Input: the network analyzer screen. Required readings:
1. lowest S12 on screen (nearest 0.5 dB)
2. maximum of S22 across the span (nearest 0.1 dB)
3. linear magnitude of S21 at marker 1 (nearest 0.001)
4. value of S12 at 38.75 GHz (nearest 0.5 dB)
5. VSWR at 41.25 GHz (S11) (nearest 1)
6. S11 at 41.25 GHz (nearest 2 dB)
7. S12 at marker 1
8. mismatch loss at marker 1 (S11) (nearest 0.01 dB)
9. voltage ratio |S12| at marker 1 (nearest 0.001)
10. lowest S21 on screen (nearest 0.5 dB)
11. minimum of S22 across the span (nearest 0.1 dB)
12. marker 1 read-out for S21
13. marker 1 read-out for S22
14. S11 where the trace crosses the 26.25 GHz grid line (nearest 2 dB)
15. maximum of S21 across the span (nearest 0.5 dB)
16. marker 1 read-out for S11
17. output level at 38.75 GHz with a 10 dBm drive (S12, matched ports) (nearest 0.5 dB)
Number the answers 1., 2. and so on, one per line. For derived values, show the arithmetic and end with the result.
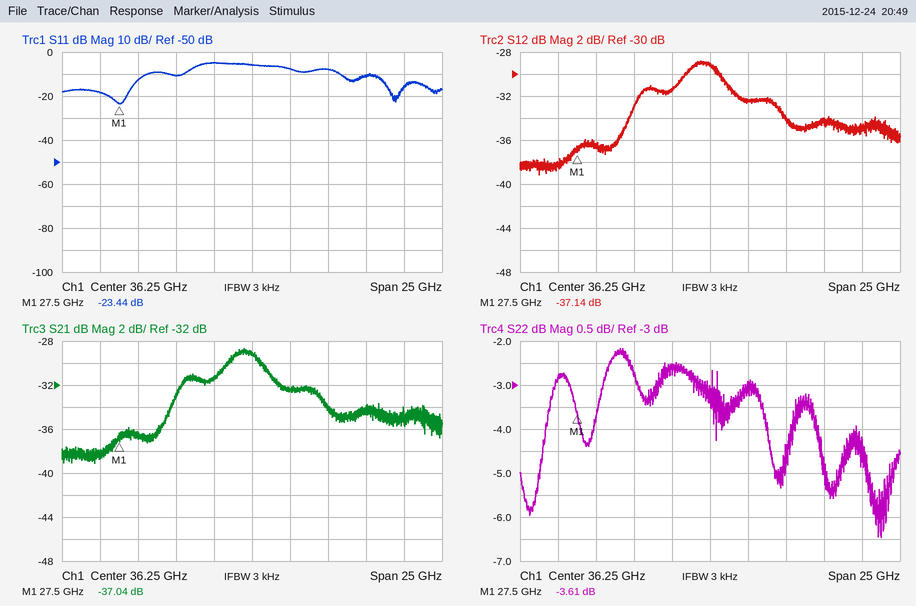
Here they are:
1. -39.0 dB
2. -2.2 dB
3. 10^(-37.04/20) ≈ 0.014
4. -32.5 dB
5. |Γ| = 10^(-8/20) = 0.3981; VSWR = (1 + 0.3981)/(1 − 0.3981) ≈ 2
6. -8 dB
7. -37.14 dB
8. −10 log10(1 − 10^(-23.44/10)) ≈ 0.02 dB
9. 10^(-37.14/20) ≈ 0.014
10. -39.0 dB
11. -6.5 dB
12. -37.04 dB
13. -3.61 dB
14. -18 dB
15. -28.5 dB
16. -23.44 dB
17. 10 dBm + (-32.5 dB) = -22.5 dBm
